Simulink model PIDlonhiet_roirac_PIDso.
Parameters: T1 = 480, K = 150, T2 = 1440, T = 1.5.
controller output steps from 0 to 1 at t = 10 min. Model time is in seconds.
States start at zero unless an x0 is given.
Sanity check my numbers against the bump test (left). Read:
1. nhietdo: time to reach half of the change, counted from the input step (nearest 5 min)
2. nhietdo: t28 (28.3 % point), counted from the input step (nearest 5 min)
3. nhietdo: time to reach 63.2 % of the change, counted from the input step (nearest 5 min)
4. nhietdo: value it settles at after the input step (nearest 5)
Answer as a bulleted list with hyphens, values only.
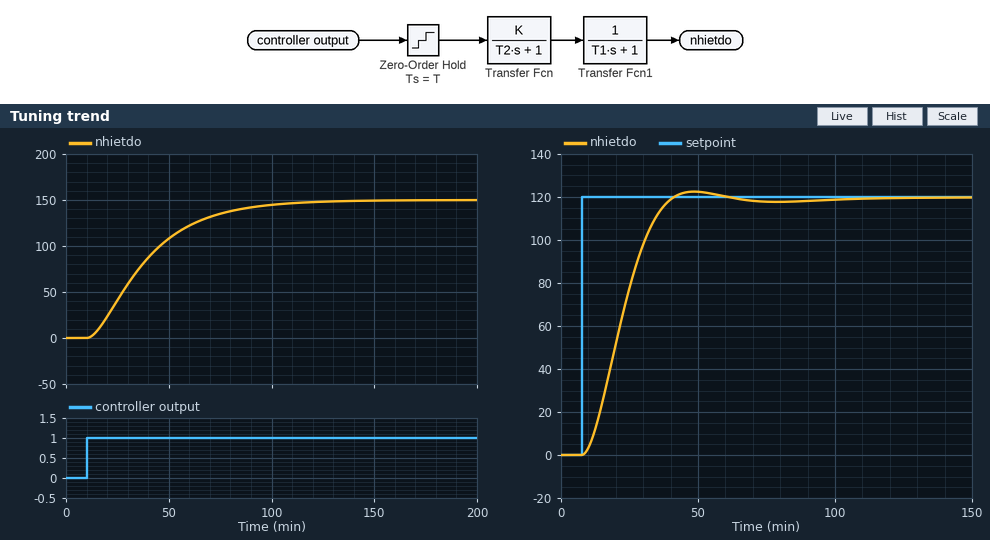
- 25 min
- 15 min
- 35 min
- 150
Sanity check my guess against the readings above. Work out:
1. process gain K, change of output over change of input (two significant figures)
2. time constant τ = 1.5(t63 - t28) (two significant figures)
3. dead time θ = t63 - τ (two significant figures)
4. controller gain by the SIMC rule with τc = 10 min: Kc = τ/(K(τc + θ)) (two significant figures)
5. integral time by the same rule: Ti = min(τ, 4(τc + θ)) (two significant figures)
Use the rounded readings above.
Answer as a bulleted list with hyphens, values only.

- 150
- 30 min
- 5.0 min
- 0.013
- 30 min
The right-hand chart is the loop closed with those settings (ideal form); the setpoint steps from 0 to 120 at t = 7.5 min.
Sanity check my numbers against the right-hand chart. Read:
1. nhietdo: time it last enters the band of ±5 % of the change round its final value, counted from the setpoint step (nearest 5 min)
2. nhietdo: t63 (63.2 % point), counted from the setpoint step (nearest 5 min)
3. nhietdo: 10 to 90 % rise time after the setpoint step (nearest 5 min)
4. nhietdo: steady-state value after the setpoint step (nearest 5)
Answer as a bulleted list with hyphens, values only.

- 30 min
- 15 min
- 20 min
- 120
